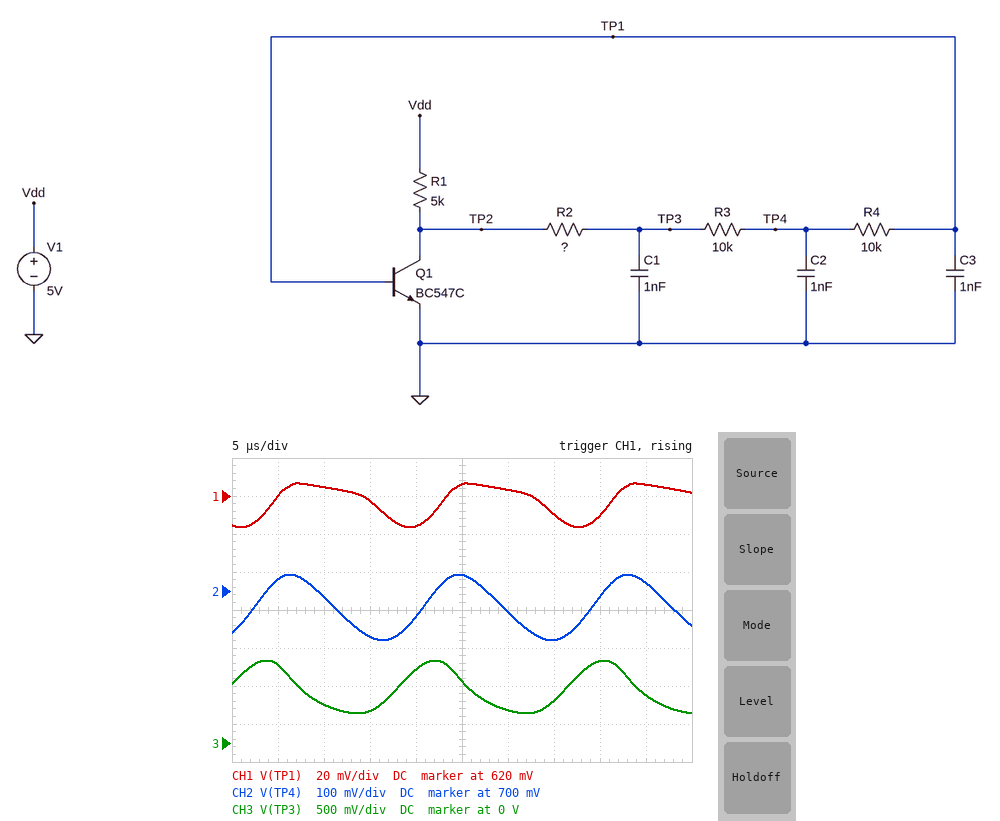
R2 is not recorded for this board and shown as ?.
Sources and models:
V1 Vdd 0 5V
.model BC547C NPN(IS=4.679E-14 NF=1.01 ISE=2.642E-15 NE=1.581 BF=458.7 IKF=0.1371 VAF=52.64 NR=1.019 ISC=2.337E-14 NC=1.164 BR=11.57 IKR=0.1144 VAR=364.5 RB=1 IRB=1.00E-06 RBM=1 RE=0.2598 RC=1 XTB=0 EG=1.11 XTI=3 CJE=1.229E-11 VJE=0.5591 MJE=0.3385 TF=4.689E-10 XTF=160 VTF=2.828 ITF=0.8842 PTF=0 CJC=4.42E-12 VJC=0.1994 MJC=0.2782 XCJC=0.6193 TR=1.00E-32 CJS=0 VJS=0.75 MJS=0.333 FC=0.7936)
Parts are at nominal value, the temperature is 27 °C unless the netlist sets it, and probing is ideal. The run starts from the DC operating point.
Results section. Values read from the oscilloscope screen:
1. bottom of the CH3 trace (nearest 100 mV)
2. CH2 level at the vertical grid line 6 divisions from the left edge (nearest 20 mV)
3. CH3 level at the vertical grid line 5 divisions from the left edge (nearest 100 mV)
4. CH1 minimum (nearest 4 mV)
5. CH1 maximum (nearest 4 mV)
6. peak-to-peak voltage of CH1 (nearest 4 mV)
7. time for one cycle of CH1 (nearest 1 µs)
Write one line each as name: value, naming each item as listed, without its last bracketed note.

bottom of the CH3 trace: 400 mV
CH2 level at the vertical grid line 6 divisions from the left edge: 640 mV
CH3 level at the vertical grid line 5 divisions from the left edge: 800 mV
CH1 minimum: 604 mV
CH1 maximum: 628 mV
peak-to-peak voltage of CH1: 24 mV
time for one cycle of CH1: 18 µs
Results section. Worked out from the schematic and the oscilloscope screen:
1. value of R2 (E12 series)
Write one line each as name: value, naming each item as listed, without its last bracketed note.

value of R2: 5.6 kΩ
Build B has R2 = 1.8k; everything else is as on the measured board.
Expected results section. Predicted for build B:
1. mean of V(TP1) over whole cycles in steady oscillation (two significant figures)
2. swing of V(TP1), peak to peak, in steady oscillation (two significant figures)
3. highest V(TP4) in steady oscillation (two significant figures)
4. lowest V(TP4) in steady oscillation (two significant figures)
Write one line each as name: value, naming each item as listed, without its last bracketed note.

mean of V(TP1) over whole cycles in steady oscillation: 620 mV
swing of V(TP1), peak to peak, in steady oscillation: 31 mV
highest V(TP4) in steady oscillation: 780 mV
lowest V(TP4) in steady oscillation: 550 mV
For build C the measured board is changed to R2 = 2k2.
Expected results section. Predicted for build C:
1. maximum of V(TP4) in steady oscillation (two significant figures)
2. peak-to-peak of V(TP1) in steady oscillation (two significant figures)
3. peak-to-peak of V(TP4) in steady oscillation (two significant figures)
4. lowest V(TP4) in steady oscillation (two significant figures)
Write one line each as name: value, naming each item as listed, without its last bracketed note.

maximum of V(TP4) in steady oscillation: 780 mV
peak-to-peak of V(TP1) in steady oscillation: 30 mV
peak-to-peak of V(TP4) in steady oscillation: 230 mV
lowest V(TP4) in steady oscillation: 550 mV
